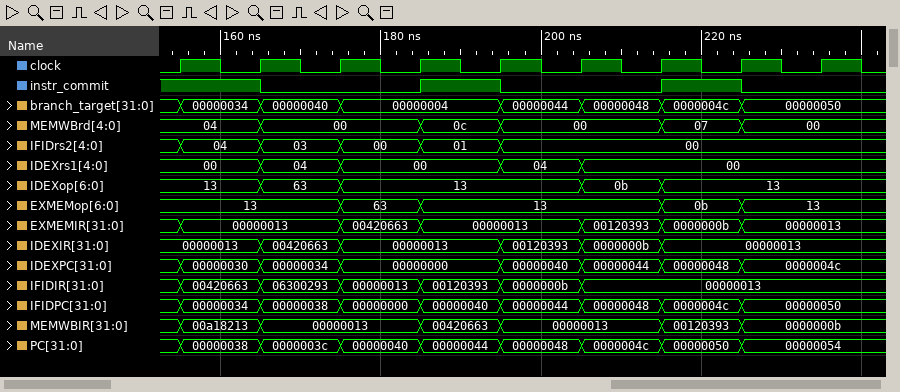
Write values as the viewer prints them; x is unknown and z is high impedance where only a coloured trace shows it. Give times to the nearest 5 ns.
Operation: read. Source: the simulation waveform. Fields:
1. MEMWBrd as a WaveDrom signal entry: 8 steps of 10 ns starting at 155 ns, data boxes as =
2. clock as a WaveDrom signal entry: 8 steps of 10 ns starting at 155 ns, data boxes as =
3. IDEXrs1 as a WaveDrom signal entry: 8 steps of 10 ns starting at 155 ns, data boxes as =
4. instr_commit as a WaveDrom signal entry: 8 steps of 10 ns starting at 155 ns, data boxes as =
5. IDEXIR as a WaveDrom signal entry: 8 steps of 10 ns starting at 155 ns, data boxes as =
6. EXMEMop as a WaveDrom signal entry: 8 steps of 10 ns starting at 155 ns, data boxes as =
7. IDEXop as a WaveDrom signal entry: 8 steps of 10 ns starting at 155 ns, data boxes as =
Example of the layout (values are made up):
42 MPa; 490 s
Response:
{name: 'MEMWBrd', wave: '==.==.==', data: '04 00 0c 00 07 00'}; {name: 'clock', wave: 'p.......'}; {name: 'IDEXrs1', wave: '===.==..', data: '00 04 00 04 00'}; {name: 'instr_commit', wave: '10.10.10'}; {name: 'IDEXIR', wave: '===.===.', data: '00000013 00420663 00000013 00120393 0000000b 00000013'}; {name: 'EXMEMop', wave: '=.==..==', data: '13 63 13 0b 13'}; {name: 'IDEXop', wave: '===..==.', data: '13 63 13 0b 13'}
